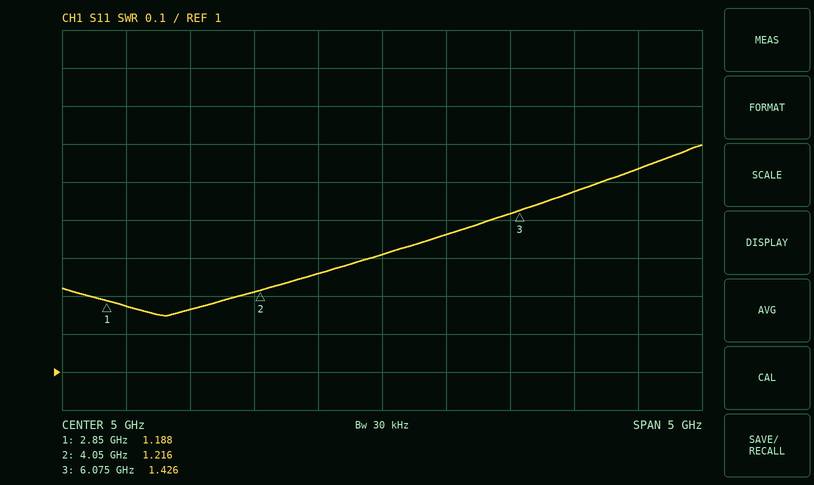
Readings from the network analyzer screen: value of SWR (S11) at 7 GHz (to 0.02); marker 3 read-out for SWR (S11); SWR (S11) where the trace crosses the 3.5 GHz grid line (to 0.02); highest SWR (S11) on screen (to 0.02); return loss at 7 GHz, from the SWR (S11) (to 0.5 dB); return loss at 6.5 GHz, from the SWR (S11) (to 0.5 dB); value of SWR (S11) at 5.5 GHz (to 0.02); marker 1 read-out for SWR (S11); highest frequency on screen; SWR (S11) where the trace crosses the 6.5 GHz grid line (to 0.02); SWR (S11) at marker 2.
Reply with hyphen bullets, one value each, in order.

- 1.54
- 1.426
- 1.16
- 1.60
- 13.5 dB
- 14.5 dB
- 1.36
- 1.188
- 7.5 GHz
- 1.48
- 1.216
